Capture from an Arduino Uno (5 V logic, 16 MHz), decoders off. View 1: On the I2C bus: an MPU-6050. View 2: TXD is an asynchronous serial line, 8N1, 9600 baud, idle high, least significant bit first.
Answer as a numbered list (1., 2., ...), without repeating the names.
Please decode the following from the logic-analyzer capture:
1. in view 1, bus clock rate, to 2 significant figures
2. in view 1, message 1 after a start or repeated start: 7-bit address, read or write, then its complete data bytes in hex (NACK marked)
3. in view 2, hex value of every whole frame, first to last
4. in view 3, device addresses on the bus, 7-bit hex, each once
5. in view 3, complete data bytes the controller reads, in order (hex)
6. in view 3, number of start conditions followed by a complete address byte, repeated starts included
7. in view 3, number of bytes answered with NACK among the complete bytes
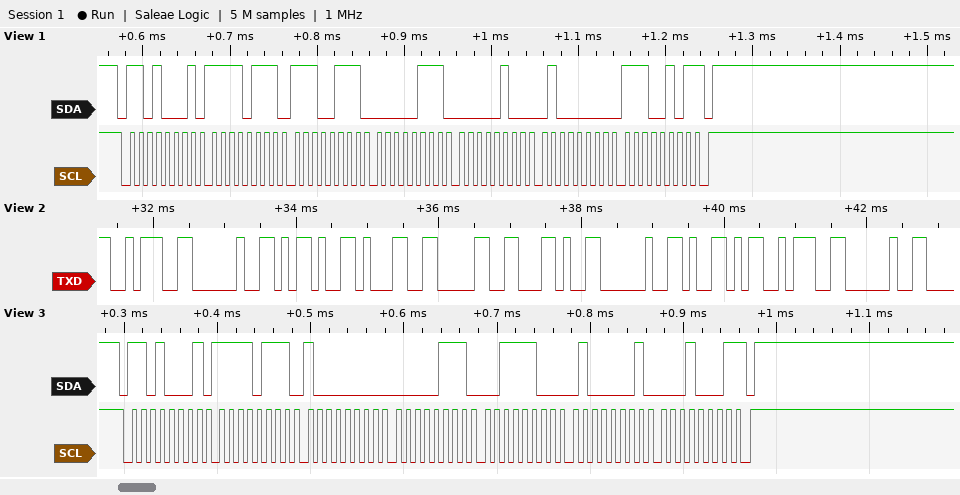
1. 100 kHz
2. 0x68 read: F7 E7 07 04 40 E5 NACK
3. 3A 20 2D 31 30 2C 20 59 3A 20
4. 0x68
5. F7 80 07 3C 41 11
6. 1
7. 1
